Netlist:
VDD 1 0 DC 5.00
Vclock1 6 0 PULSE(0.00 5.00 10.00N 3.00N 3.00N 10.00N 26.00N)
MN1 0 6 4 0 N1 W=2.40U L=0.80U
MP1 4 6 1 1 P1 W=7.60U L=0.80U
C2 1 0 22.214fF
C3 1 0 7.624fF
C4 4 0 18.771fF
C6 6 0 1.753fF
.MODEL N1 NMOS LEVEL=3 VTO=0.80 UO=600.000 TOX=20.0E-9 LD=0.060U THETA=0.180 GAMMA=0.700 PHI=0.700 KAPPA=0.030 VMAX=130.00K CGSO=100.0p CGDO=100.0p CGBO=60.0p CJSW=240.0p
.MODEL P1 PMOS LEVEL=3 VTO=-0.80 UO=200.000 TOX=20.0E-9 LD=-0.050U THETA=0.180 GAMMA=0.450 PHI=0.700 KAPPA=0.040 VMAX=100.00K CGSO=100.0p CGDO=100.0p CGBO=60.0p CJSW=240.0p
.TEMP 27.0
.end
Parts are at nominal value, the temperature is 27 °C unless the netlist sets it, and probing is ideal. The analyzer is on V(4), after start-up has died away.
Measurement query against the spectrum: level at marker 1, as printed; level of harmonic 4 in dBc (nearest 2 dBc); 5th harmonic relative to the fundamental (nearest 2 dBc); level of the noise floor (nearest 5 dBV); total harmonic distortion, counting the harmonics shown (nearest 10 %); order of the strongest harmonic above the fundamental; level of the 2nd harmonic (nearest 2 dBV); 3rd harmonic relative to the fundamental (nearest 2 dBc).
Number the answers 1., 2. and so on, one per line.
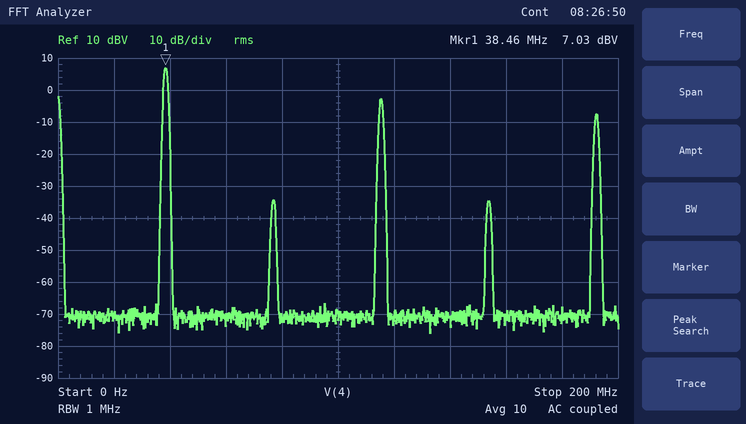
1. 7.03 dBV
2. -42 dBc
3. -14 dBc
4. -70 dBV
5. 40 %
6. 3
7. -34 dBV
8. -10 dBc
